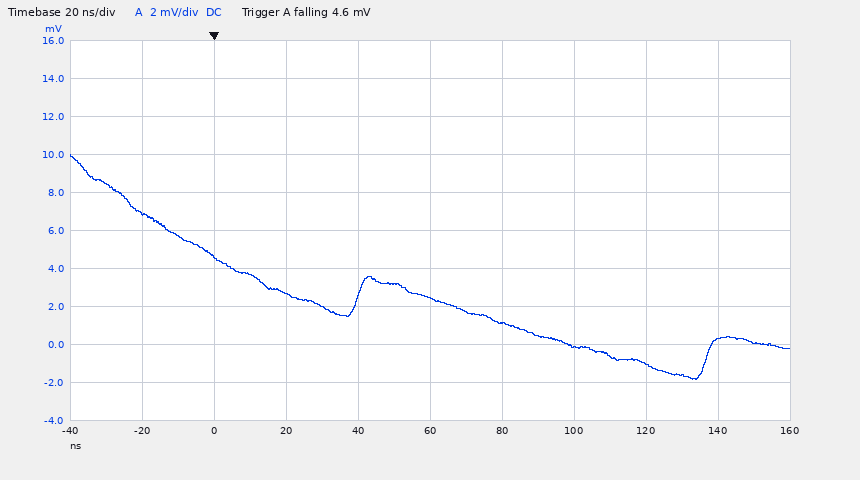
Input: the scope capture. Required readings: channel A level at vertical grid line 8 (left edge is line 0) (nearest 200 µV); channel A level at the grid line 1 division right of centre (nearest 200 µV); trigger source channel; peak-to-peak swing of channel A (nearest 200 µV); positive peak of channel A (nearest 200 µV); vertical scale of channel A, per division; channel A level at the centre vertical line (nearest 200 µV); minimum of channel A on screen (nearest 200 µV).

-1.0 mV
1.2 mV
channel A
11.8 mV
10.0 mV
2 mV
2.4 mV
-1.8 mV
